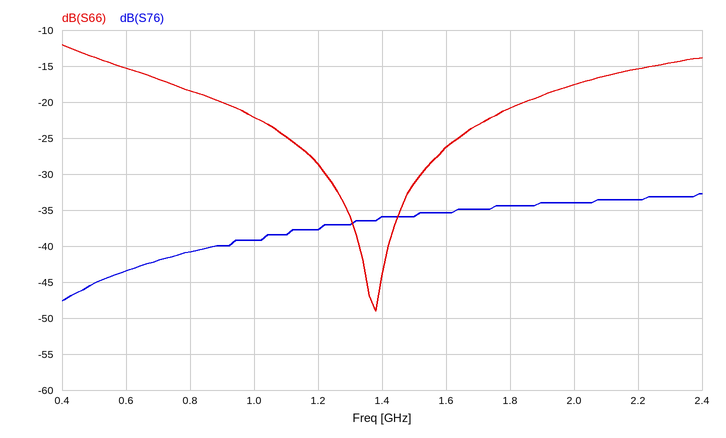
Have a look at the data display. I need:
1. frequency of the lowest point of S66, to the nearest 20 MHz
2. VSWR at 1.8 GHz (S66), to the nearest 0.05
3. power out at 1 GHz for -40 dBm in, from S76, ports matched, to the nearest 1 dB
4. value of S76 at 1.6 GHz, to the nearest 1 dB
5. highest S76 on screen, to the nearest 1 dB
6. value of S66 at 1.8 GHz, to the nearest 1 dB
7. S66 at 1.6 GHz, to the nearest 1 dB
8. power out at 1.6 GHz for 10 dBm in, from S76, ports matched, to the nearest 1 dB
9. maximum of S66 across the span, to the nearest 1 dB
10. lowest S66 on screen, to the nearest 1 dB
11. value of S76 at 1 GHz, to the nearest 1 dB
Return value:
1.38 GHz
1.20
-79 dBm
-35 dB
-33 dB
-21 dB
-26 dB
-25 dBm
-12 dB
-49 dB
-39 dB
